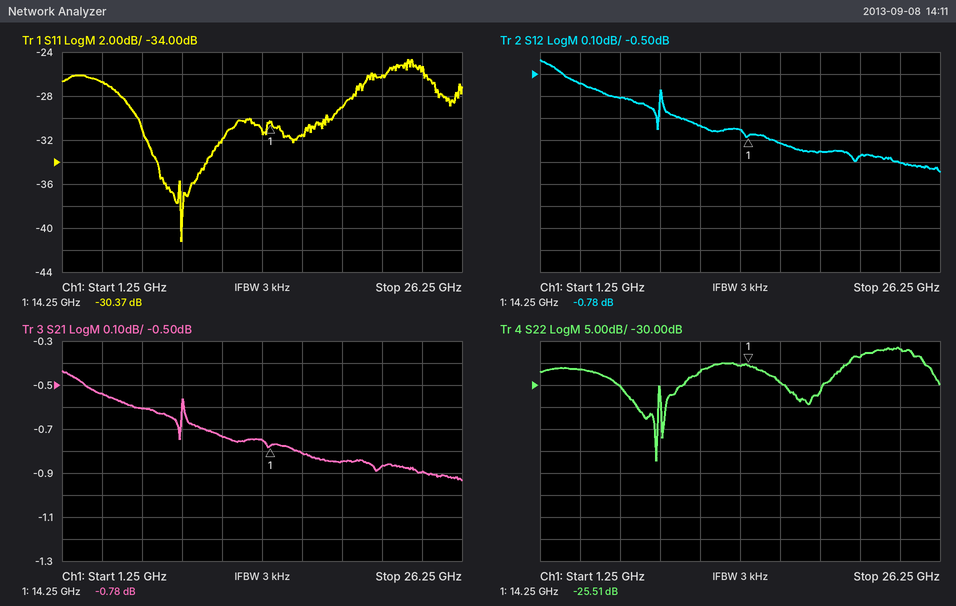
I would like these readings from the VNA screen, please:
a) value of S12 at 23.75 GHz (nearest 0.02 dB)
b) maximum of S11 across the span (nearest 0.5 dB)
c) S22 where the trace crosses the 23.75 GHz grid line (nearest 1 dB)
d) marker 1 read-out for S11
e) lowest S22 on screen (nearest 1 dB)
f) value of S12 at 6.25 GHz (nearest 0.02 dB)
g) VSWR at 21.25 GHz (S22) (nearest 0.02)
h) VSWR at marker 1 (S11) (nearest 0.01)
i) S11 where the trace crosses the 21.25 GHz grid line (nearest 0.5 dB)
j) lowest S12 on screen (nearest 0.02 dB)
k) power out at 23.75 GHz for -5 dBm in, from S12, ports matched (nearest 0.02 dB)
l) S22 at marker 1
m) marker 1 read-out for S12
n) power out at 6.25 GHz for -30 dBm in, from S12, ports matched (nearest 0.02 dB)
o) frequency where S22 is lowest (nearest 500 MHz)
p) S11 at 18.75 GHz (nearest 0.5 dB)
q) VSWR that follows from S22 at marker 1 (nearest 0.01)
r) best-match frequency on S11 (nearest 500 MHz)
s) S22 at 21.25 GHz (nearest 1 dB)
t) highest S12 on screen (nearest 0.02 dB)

-0.90 dB
-24.5 dB
-22 dB
-30.37 dB
-47 dB
-0.60 dB
1.14
1.06
-26.0 dB
-0.94 dB
-5.90 dBm
-25.51 dB
-0.78 dB
-30.60 dBm
8.5 GHz
-29.0 dB
1.11
8.5 GHz
-24 dB
-0.44 dB
